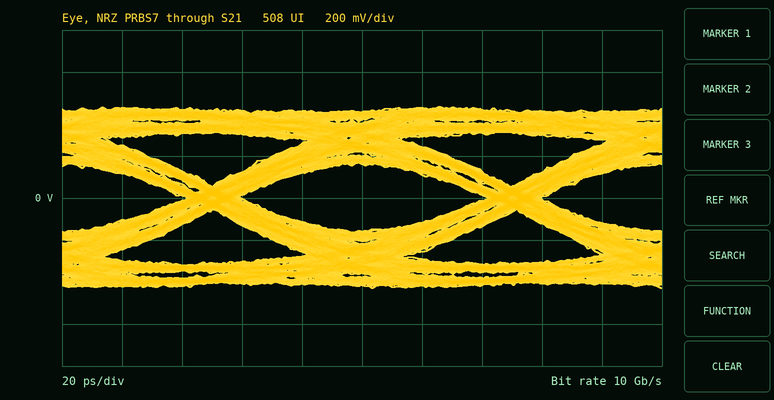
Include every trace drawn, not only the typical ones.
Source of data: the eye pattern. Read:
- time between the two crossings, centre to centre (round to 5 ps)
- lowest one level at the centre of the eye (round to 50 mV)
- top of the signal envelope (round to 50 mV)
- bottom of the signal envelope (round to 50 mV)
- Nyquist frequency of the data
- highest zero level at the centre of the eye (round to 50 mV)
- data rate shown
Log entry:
100 ps
150 mV
450 mV
-450 mV
5 GHz
-150 mV
10 Gb/s
